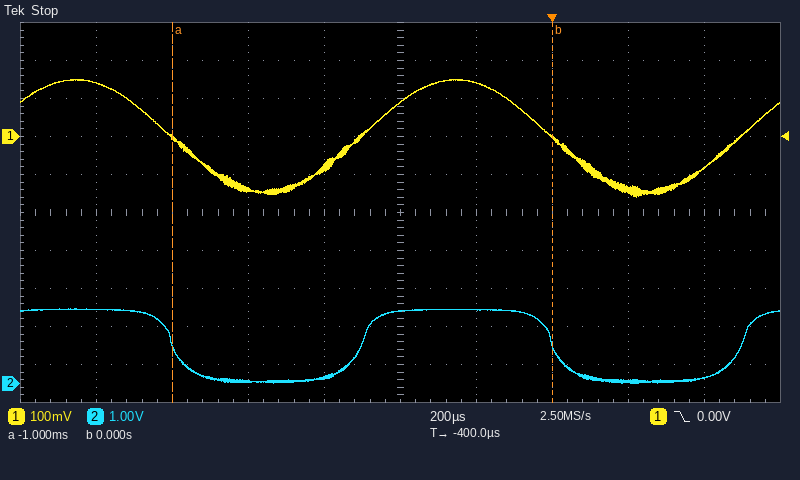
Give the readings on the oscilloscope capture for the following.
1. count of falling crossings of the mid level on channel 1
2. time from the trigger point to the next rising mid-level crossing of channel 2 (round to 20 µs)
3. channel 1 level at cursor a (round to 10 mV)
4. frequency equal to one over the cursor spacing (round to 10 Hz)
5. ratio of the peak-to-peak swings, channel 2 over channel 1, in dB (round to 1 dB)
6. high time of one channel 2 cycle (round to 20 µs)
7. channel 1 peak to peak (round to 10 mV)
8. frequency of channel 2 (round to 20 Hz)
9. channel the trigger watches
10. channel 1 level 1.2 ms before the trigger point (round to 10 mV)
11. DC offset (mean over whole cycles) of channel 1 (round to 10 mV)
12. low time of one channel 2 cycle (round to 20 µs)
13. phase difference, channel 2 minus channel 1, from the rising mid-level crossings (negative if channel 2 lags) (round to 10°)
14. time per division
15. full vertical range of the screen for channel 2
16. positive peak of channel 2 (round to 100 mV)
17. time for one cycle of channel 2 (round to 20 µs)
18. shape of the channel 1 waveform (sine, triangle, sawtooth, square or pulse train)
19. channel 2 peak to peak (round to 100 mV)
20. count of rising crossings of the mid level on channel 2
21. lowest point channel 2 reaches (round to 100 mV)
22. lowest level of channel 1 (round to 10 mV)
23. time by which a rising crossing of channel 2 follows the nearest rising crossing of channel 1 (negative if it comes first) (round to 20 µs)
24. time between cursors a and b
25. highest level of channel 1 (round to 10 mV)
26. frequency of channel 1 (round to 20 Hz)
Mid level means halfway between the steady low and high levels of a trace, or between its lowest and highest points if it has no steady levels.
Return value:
2
500 µs
0 mV
1.00 kHz
16 dB
500 µs
310 mV
1.00 kHz
channel 1
140 mV
0 mV
500 µs
0°
200 µs
10 V
2.0 V
1.00 ms
sine
2.0 V
2
0.0 V
-160 mV
0 µs
1.00 ms
150 mV
1.00 kHz
